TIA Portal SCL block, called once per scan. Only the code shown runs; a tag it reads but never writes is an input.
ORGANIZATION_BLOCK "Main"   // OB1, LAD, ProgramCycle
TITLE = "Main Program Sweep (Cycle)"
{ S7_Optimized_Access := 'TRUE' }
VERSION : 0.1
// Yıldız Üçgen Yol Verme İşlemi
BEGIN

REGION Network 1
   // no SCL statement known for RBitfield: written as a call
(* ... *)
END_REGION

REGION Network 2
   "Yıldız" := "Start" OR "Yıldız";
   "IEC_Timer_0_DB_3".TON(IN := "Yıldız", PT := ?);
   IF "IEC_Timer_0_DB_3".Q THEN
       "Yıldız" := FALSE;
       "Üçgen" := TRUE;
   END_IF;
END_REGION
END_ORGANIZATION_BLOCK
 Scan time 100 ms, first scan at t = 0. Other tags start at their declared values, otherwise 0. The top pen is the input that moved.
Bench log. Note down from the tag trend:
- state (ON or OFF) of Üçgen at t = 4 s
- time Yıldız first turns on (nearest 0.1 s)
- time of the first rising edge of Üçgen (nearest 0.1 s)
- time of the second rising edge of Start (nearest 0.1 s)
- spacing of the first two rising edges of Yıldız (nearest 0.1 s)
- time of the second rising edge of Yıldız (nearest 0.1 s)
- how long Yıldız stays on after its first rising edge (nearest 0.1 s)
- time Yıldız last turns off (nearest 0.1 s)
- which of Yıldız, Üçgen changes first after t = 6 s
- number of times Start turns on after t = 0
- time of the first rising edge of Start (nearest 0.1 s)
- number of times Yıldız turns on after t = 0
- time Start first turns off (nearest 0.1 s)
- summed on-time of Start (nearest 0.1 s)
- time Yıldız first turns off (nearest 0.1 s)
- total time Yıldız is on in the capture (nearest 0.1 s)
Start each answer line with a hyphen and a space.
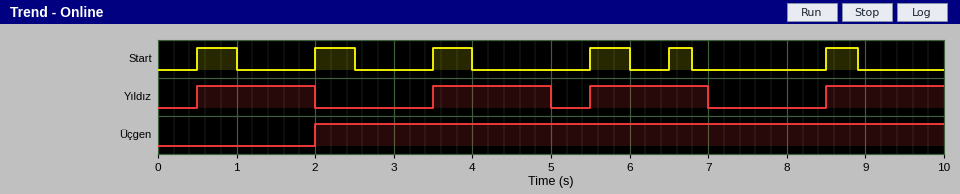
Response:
- ON
- 0.5 s
- 2.0 s
- 2.0 s
- 3.0 s
- 3.5 s
- 1.5 s
- 7.0 s
- Yıldız
- 6
- 0.5 s
- 4
- 1.0 s
- 2.7 s
- 2.0 s
- 6.0 s
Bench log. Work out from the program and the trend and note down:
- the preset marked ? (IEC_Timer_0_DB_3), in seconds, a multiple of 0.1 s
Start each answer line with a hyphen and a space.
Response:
- 1.5 s
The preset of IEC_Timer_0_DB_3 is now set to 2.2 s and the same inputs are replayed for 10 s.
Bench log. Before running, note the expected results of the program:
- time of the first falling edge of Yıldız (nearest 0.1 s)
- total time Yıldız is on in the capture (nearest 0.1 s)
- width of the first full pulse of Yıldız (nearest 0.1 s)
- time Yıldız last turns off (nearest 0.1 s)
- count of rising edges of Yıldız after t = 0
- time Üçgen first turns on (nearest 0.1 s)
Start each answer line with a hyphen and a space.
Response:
- 2.7 s
- 6.6 s
- 2.2 s
- 8.7 s
- 3
- 2.7 s
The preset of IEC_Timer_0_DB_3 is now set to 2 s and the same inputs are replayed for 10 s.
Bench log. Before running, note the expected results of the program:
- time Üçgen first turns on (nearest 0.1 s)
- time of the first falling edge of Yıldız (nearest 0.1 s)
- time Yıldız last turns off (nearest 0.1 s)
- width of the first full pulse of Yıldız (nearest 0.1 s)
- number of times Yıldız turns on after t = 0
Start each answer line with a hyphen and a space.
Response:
- 2.5 s
- 2.5 s
- 8.5 s
- 2.0 s
- 3
